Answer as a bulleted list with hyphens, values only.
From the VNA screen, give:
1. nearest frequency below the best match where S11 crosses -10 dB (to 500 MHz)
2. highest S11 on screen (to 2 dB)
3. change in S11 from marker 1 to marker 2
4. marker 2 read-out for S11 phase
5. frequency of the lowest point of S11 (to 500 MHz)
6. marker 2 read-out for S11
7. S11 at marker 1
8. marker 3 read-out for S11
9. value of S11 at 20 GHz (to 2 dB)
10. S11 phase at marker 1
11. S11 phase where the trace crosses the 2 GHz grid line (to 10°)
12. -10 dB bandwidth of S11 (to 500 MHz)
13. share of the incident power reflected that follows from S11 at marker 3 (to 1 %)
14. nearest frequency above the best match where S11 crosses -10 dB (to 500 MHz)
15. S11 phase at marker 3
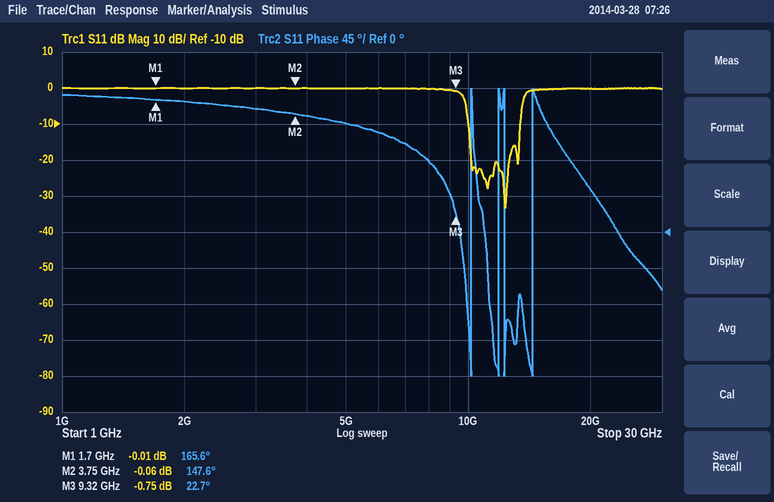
- 10.0 GHz
- 0 dB
- -0.05 dB
- 147.6°
- 12.5 GHz
- -0.06 dB
- -0.01 dB
- -0.75 dB
- 0 dB
- 165.6°
- 160°
- 3.5 GHz
- 84 %
- 13.5 GHz
- 22.7°
